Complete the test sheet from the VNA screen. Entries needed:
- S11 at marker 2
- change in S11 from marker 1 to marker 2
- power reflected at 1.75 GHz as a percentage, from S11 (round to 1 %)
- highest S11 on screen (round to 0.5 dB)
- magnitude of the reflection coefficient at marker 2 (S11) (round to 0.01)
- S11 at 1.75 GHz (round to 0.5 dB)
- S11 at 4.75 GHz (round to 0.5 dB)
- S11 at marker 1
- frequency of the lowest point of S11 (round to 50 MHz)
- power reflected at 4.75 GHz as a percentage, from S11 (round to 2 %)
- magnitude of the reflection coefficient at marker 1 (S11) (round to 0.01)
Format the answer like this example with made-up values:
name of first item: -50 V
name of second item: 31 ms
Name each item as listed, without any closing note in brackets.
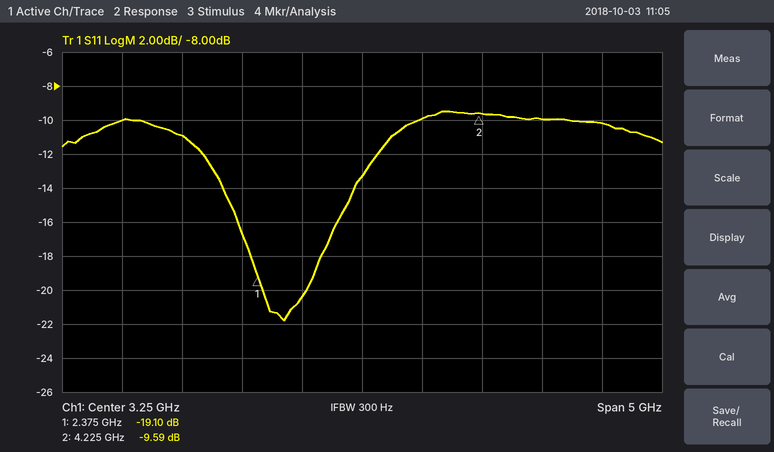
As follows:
S11 at marker 2: -9.59 dB
change in S11 from marker 1 to marker 2: 9.51 dB
power reflected at 1.75 GHz as a percentage, from S11: 8 %
highest S11 on screen: -9.5 dB
magnitude of the reflection coefficient at marker 2 (S11): 0.33
S11 at 1.75 GHz: -11.0 dB
S11 at 4.75 GHz: -10.0 dB
S11 at marker 1: -19.10 dB
frequency of the lowest point of S11: 2.60 GHz
power reflected at 4.75 GHz as a percentage, from S11: 10 %
magnitude of the reflection coefficient at marker 1 (S11): 0.11
